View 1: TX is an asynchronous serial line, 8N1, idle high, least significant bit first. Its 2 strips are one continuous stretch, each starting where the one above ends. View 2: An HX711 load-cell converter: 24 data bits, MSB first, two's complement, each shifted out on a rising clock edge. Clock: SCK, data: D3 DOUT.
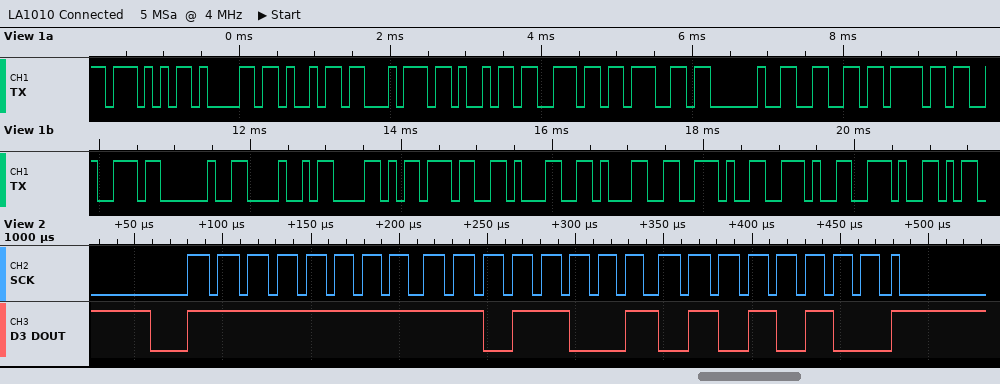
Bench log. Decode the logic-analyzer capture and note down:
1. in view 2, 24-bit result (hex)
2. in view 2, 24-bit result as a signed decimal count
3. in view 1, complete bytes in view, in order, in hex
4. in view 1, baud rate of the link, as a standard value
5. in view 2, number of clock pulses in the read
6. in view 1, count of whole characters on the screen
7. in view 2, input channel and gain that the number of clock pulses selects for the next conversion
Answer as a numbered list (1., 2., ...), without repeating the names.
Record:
1. 0xFFD954
2. -9900
3. 0x57 0x61 0x69 0x74 0x69 0x6E 0x67 0x20 0x66 0x6F 0x72 0x20 0x48 0x58 0x37 0x31 0x31 0x2E 0x2E 0x2E
4. 9600 baud
5. 25
6. 20
7. channel A, gain 128
